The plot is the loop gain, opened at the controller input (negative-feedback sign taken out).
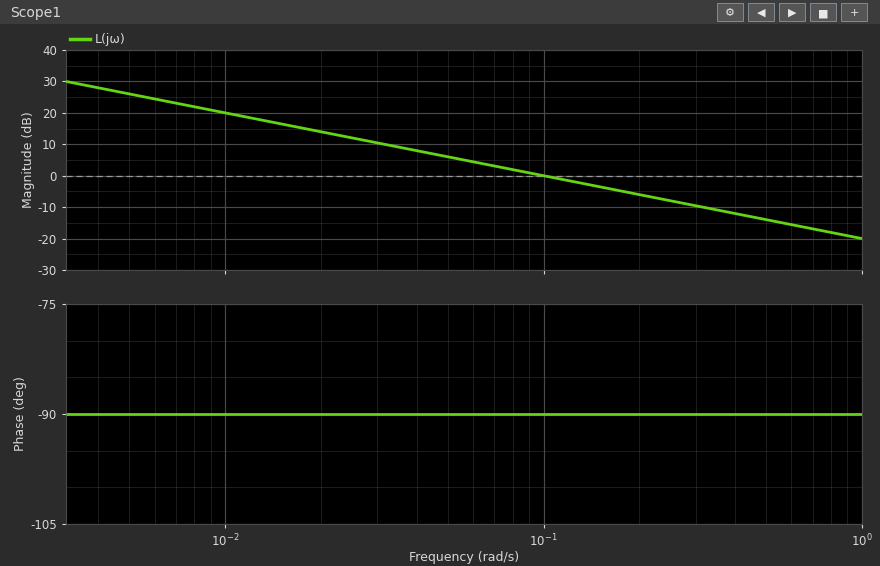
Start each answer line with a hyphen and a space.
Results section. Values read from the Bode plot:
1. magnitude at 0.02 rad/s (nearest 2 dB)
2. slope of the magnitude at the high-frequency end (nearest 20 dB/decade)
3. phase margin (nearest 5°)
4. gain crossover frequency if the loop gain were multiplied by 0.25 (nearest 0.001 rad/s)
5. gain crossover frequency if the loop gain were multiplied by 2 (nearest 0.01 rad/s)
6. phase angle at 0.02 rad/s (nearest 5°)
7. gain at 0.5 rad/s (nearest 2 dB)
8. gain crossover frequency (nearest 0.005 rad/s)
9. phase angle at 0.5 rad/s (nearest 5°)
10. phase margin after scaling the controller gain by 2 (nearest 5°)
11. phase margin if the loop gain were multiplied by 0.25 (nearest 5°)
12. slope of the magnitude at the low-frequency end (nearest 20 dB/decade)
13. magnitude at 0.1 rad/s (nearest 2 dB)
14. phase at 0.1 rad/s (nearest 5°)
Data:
- 14 dB
- -20 dB/decade
- 90°
- 0.025 rad/s
- 0.20 rad/s
- -90°
- -14 dB
- 0.100 rad/s
- -90°
- 90°
- 90°
- -20 dB/decade
- 0 dB
- -90°
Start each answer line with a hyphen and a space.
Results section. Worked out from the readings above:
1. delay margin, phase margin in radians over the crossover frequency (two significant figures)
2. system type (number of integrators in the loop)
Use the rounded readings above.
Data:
- 16 s
- 1
